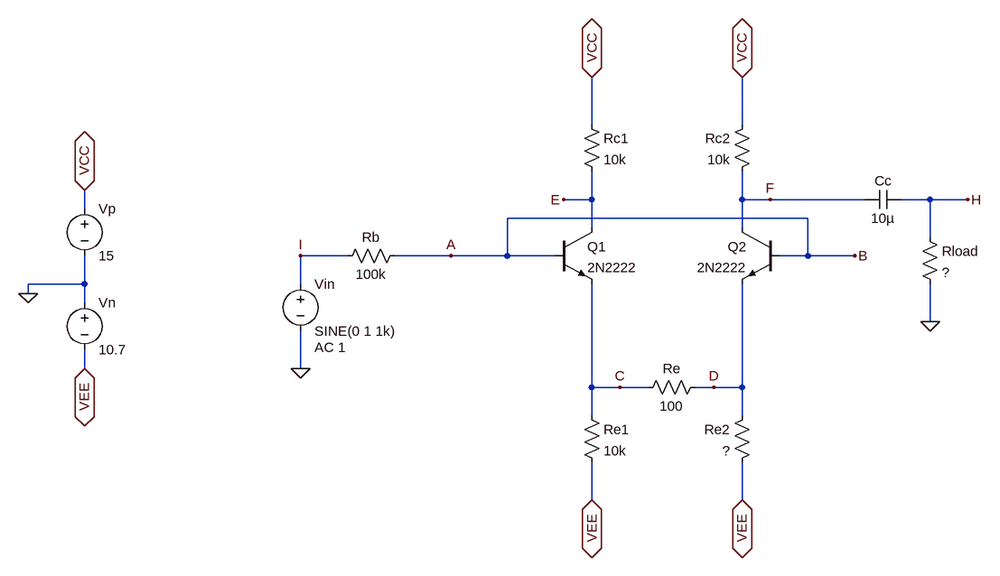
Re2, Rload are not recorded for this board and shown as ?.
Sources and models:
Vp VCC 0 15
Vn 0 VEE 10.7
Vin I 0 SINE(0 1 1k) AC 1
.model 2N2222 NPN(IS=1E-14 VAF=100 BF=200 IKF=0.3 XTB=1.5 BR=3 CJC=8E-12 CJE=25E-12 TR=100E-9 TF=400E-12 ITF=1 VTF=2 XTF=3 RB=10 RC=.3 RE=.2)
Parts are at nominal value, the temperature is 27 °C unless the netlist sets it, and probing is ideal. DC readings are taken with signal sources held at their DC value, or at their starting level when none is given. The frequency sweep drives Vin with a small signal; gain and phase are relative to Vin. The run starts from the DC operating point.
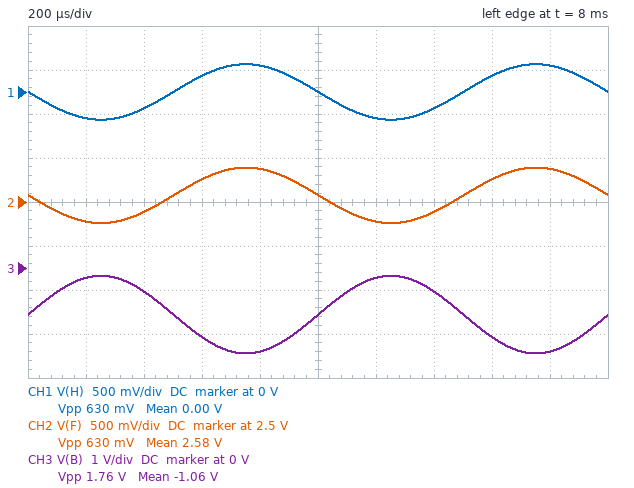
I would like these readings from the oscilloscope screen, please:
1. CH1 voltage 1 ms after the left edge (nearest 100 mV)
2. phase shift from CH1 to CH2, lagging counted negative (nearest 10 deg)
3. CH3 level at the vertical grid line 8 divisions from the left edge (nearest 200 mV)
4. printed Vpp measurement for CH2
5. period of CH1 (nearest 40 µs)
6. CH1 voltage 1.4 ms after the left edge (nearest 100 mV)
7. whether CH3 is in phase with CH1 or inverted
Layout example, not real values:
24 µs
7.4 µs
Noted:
0 V
0 deg
-1.6 V
630 mV
1.00 ms
-200 mV
inverted
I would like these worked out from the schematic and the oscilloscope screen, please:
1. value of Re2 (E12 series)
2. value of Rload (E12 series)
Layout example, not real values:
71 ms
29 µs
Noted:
6.8 kΩ
3.3 kΩ
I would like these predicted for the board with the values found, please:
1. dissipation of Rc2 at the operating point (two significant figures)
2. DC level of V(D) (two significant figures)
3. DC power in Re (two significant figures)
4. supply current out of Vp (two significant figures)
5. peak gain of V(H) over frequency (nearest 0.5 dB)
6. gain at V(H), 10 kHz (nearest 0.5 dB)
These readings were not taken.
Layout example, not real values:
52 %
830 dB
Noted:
15 mW
-1.7 V
530 nW
2.2 mA
-10.0 dB
-10.0 dB
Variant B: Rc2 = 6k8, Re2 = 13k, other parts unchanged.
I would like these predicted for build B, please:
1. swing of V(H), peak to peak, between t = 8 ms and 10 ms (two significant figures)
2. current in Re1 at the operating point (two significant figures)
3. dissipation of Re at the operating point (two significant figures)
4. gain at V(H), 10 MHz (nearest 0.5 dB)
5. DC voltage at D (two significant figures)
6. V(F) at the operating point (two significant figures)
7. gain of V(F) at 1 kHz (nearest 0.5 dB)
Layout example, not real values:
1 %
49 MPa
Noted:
320 mV
930 µA
220 nW
-38.5 dB
-1.4 V
9.8 V
-16.0 dB
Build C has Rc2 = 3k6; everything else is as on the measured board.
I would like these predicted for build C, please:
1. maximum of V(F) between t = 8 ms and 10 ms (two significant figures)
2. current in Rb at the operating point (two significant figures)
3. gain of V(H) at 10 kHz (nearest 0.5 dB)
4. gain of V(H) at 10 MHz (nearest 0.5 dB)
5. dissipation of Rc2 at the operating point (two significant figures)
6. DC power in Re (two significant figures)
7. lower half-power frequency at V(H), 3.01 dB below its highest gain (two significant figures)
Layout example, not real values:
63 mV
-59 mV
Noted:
11 V
10 µA
-13.0 dB
-39.5 dB
5.7 mW
360 nW
2.3 Hz
